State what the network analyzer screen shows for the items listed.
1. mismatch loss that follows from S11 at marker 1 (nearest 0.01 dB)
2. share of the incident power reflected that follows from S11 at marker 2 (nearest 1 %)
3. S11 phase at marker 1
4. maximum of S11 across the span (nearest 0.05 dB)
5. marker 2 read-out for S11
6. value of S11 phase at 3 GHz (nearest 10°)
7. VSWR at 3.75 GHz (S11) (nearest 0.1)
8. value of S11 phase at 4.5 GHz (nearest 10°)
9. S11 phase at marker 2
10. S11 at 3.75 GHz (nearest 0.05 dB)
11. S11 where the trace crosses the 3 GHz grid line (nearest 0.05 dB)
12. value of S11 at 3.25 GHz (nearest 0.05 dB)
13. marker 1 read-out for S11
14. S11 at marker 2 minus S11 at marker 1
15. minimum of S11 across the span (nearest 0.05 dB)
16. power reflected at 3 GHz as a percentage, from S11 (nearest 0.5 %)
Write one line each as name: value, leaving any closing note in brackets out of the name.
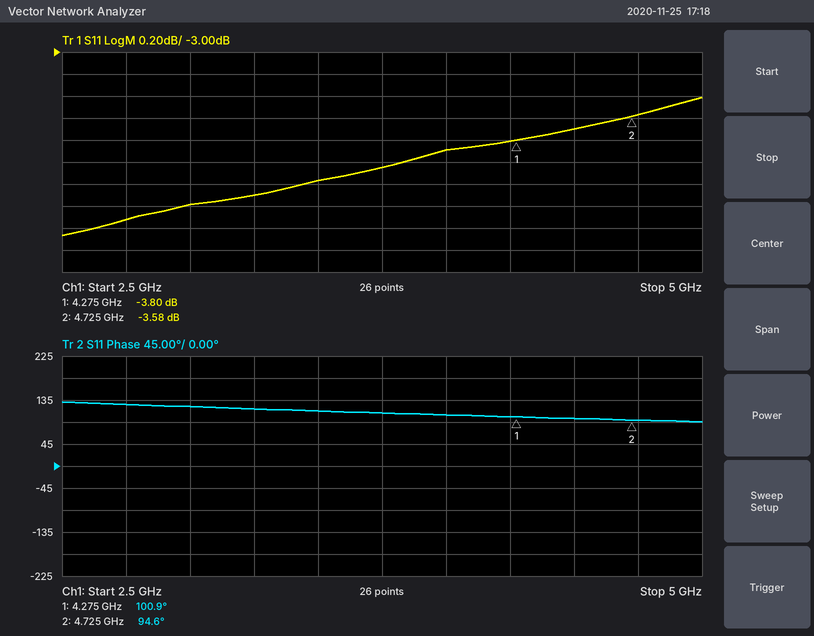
mismatch loss that follows from S11 at marker 1: 2.34 dB
share of the incident power reflected that follows from S11 at marker 2: 44 %
S11 phase at marker 1: 100.9°
maximum of S11 across the span: -3.40 dB
marker 2 read-out for S11: -3.58 dB
value of S11 phase at 3 GHz: 120°
VSWR at 3.75 GHz (S11): 4.4
value of S11 phase at 4.5 GHz: 100°
S11 phase at marker 2: 94.6°
S11 at 3.75 GHz: -4.05 dB
S11 where the trace crosses the 3 GHz grid line: -4.40 dB
value of S11 at 3.25 GHz: -4.30 dB
marker 1 read-out for S11: -3.80 dB
S11 at marker 2 minus S11 at marker 1: 0.22 dB
minimum of S11 across the span: -4.65 dB
power reflected at 3 GHz as a percentage, from S11: 36.5 %
